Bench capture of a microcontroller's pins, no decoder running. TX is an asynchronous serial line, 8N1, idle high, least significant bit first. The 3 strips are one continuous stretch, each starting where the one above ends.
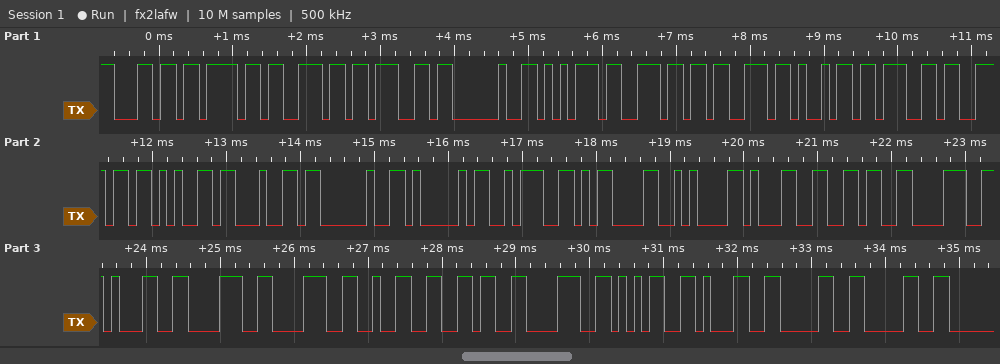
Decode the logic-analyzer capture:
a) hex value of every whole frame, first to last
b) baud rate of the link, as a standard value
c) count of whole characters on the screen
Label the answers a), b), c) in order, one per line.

a) 0x6C 0x6F 0x6E 0x67 0x20 0x75 0x6E 0x73 0x69 0x67 0x6E 0x65 0x64 0x20 0x41 0x3A 0x0D 0x0A 0x31 0x36 0x38 0x31 0x38 0x38 0x32 0x36 0x38 0x35 0x31 0x30 0x30
b) 9600 baud
c) 31
